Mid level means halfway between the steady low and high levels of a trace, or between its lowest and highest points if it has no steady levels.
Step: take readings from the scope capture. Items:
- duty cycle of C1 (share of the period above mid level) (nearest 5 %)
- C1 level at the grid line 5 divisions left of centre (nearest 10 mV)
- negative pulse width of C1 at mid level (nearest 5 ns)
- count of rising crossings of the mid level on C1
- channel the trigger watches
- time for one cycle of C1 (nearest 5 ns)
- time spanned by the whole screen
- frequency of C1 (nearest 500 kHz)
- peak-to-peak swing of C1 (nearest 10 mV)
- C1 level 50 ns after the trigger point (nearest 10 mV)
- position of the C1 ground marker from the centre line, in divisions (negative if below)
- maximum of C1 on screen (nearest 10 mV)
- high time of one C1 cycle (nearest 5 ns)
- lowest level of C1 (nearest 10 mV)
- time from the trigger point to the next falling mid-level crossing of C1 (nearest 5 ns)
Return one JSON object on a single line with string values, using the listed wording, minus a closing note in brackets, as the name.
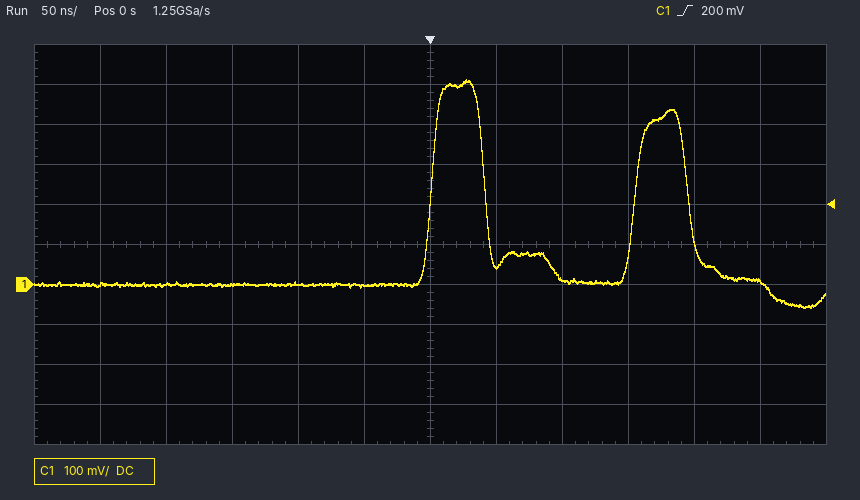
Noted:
{"duty cycle of C1 (share of the period above mid level)": "25 %", "C1 level at the grid line 5 divisions left of centre": "0 mV", "negative pulse width of C1 at mid level": "115 ns", "count of rising crossings of the mid level on C1": "2", "channel the trigger watches": "C1", "time for one cycle of C1": "155 ns", "time spanned by the whole screen": "600 ns", "frequency of C1": "6.5 MHz", "peak-to-peak swing of C1": "570 mV", "C1 level 50 ns after the trigger point": "50 mV", "position of the C1 ground marker from the centre line, in divisions": "-1.0 div", "maximum of C1 on screen": "510 mV", "high time of one C1 cycle": "40 ns", "lowest level of C1": "-60 mV", "time from the trigger point to the next falling mid-level crossing of C1": "40 ns"}
